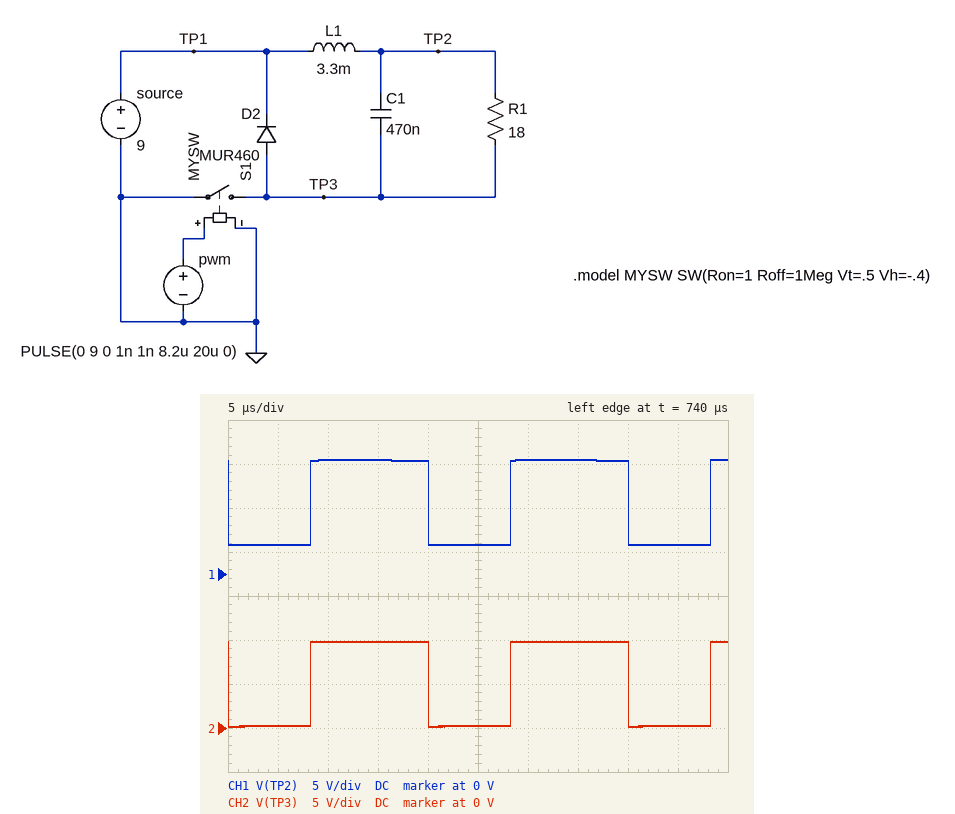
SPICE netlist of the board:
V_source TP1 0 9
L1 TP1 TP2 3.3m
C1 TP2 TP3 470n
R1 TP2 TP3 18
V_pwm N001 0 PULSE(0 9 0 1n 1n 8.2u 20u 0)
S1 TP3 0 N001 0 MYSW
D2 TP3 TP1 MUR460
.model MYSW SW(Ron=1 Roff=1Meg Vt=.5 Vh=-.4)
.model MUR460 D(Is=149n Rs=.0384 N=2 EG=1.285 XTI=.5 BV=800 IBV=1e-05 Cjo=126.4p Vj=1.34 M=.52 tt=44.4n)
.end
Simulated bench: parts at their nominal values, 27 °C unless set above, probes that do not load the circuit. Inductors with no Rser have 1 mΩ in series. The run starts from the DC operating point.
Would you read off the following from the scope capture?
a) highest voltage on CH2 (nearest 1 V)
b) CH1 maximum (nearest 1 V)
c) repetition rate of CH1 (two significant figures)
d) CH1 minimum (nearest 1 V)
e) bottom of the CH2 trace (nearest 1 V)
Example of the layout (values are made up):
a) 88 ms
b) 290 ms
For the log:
a) 10 V
b) 13 V
c) 50 kHz
d) 3 V
e) 0 V
